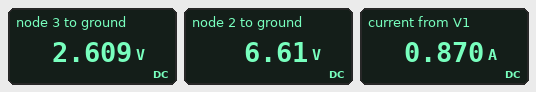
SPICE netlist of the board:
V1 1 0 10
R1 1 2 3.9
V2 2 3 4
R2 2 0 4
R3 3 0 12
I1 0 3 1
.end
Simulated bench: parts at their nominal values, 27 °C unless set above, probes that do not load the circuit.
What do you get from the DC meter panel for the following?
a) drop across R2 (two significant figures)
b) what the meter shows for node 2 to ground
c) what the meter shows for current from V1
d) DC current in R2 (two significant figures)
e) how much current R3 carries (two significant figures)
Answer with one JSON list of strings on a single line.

["6.6 V", "6.61 V", "0.870 A", "1.7 A", "220 mA"]
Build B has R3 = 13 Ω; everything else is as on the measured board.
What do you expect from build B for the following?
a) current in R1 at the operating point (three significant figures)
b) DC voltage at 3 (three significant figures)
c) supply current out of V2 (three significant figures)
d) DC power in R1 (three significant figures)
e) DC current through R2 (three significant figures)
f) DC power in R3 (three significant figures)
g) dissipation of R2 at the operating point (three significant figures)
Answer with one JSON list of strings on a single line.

["862 mA", "2.64 V", "797 mA", "2.90 W", "1.66 A", "535 mW", "11.0 W"]
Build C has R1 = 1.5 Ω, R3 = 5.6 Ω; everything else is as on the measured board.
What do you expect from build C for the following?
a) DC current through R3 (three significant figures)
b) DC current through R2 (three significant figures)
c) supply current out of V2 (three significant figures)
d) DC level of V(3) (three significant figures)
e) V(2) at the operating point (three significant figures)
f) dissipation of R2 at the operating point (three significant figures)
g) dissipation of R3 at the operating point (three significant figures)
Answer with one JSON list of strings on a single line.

["652 mA", "1.91 A", "348 mA", "3.65 V", "7.65 V", "14.6 W", "2.38 W"]
